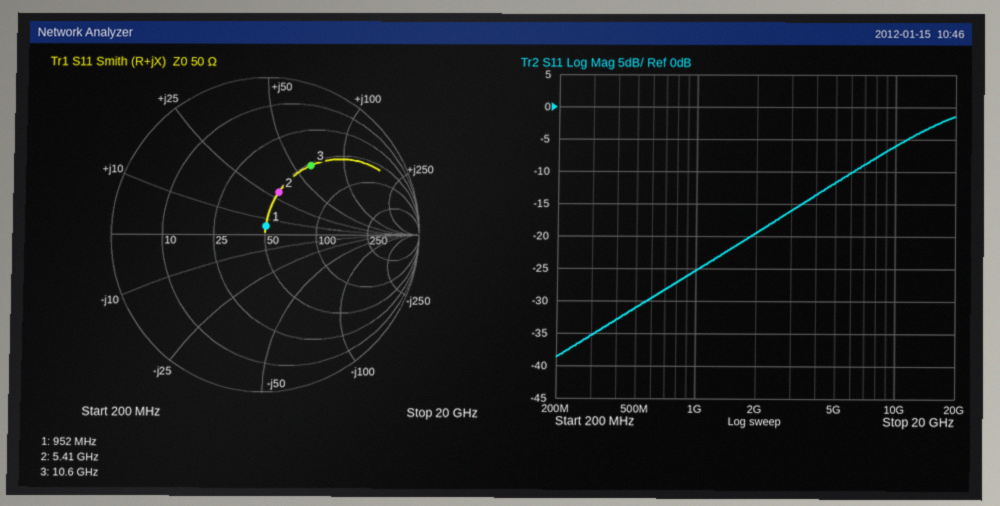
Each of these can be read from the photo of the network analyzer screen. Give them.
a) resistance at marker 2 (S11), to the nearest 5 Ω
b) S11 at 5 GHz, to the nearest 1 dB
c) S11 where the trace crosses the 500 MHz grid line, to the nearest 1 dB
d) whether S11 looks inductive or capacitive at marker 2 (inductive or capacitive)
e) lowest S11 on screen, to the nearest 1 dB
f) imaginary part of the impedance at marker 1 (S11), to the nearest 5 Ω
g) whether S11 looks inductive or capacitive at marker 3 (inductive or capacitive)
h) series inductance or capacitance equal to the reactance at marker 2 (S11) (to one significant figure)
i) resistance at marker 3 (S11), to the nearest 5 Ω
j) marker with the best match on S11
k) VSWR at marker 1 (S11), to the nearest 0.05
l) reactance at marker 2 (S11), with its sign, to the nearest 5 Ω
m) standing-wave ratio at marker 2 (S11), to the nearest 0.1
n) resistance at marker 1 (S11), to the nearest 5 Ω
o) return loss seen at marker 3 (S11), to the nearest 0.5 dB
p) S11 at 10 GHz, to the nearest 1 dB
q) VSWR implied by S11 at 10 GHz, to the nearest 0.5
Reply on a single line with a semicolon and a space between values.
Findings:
50 Ω; -12 dB; -31 dB; inductive; -39 dB; +5 Ω; inductive; 900 pH; 50 Ω; marker 1; 1.10; +30 Ω; 1.8; 50 Ω; 5.5 dB; -6 dB; 3.0
